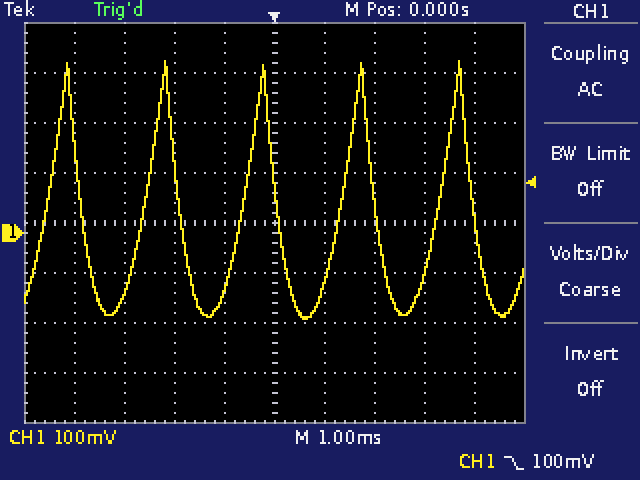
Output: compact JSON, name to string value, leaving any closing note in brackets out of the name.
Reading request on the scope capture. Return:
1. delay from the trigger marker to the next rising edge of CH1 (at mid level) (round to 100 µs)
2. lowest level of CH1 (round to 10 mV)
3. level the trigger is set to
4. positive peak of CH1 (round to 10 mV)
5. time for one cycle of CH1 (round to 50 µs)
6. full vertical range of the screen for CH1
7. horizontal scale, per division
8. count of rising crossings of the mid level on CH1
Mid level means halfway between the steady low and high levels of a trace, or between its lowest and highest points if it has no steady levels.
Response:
{"delay from the trigger marker to the next rising edge of CH1 (at mid level)": "1.4 ms", "lowest level of CH1": "-170 mV", "level the trigger is set to": "100 mV", "positive peak of CH1": "340 mV", "time for one cycle of CH1": "1.95 ms", "full vertical range of the screen for CH1": "800 mV", "horizontal scale, per division": "1 ms", "count of rising crossings of the mid level on CH1": "5"}
